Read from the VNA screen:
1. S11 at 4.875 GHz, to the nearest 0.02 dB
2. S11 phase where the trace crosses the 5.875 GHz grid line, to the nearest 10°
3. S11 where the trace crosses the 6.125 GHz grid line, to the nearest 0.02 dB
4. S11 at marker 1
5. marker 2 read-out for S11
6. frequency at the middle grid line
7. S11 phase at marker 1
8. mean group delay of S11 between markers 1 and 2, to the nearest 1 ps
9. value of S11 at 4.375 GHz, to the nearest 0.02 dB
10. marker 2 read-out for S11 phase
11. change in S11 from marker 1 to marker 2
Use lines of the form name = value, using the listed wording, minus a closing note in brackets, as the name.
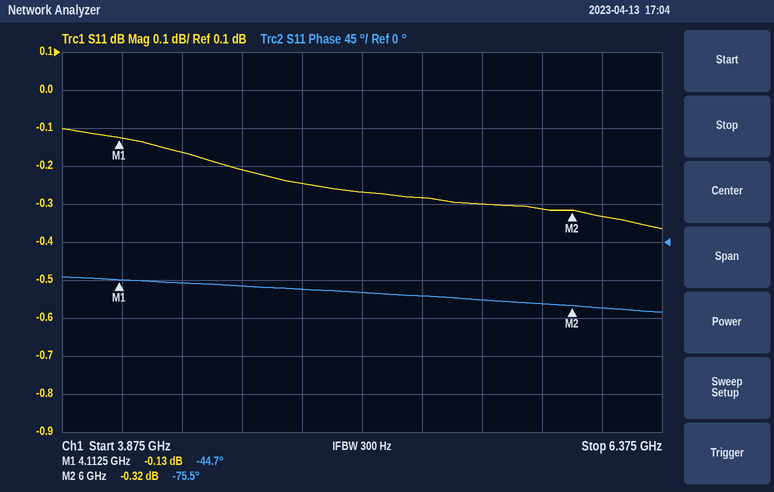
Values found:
S11 at 4.875 GHz, to the nearest 0.02 dB = -0.24 dB
S11 phase where the trace crosses the 5.875 GHz grid line, to the nearest 10° = -70°
S11 where the trace crosses the 6.125 GHz grid line, to the nearest 0.02 dB = -0.34 dB
S11 at marker 1 = -0.13 dB
marker 2 read-out for S11 = -0.32 dB
frequency at the middle grid line = 5.125 GHz
S11 phase at marker 1 = -44.7°
mean group delay of S11 between markers 1 and 2, to the nearest 1 ps = 45 ps
value of S11 at 4.375 GHz, to the nearest 0.02 dB = -0.16 dB
marker 2 read-out for S11 phase = -75.5°
change in S11 from marker 1 to marker 2 = -0.19 dB
